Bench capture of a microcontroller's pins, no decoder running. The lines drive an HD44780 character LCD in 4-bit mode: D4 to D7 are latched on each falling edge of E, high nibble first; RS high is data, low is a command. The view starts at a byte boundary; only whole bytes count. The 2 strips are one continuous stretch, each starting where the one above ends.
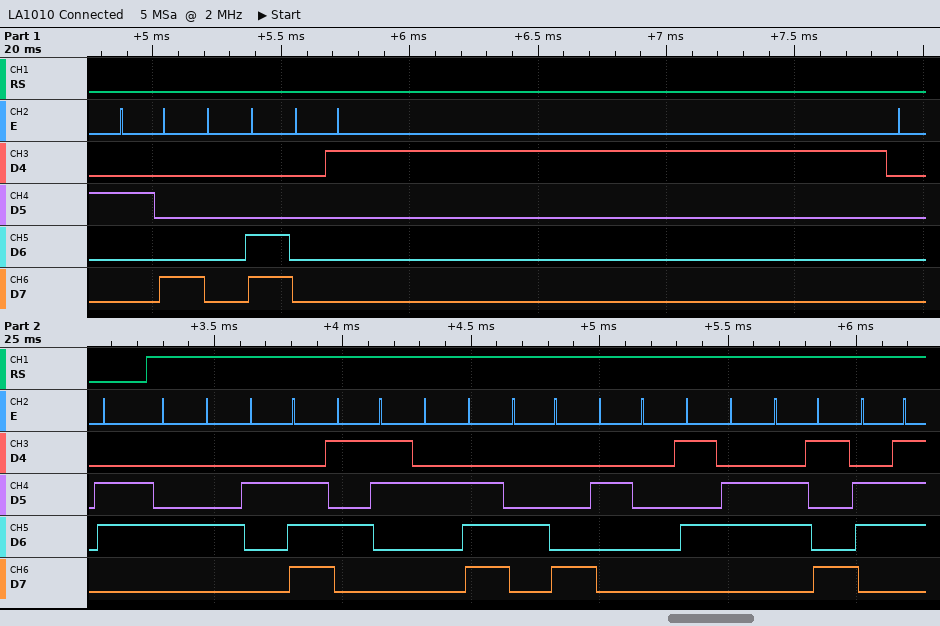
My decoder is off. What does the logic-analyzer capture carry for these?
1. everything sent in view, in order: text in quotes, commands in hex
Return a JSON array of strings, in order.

["0x28 0x0C 0x01 0x06 \"D.S.H Vig\""]
